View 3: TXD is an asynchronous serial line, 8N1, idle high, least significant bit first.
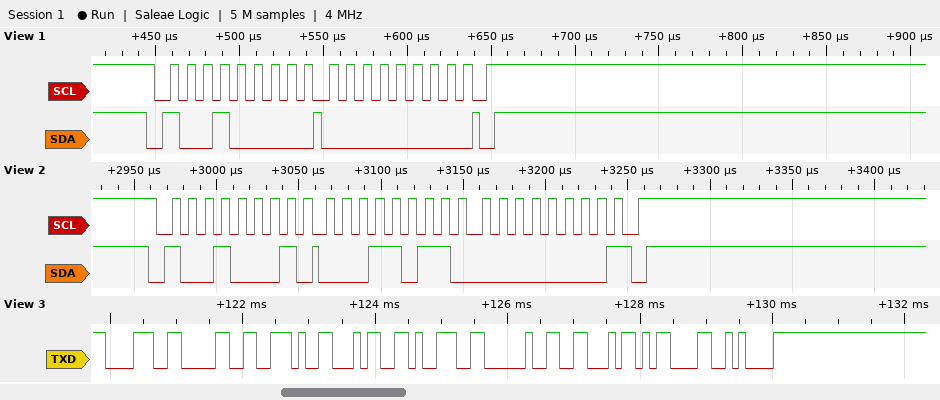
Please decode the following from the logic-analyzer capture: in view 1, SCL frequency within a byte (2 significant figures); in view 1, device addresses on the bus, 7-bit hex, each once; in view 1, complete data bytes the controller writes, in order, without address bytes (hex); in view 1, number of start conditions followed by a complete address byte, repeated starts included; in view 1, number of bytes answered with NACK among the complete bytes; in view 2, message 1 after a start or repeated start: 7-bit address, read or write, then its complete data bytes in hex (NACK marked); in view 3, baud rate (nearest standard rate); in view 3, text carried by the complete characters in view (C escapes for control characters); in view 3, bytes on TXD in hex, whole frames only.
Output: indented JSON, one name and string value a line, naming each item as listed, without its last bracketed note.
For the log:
{
  "in view 1, SCL frequency within a byte": "100 kHz",
  "in view 1, device addresses on the bus, 7-bit hex, each once": "0x48",
  "in view 1, complete data bytes the controller writes, in order, without address bytes": "00",
  "in view 1, number of start conditions followed by a complete address byte, repeated starts included": "1",
  "in view 1, number of bytes answered with NACK among the complete bytes": "0",
  "in view 2, message 1 after a start or repeated start: 7-bit address, read or write, then its complete data bytes in hex": "0x48 read: 1B 00 NACK",
  "in view 3, baud rate": "9600 baud",
  "in view 3, text carried by the complete characters in view": "\"80.49 F\\r\\n\"",
  "in view 3, bytes on TXD in hex, whole frames only": "38 30 2E 34 39 20 46 0D 0A"
}
